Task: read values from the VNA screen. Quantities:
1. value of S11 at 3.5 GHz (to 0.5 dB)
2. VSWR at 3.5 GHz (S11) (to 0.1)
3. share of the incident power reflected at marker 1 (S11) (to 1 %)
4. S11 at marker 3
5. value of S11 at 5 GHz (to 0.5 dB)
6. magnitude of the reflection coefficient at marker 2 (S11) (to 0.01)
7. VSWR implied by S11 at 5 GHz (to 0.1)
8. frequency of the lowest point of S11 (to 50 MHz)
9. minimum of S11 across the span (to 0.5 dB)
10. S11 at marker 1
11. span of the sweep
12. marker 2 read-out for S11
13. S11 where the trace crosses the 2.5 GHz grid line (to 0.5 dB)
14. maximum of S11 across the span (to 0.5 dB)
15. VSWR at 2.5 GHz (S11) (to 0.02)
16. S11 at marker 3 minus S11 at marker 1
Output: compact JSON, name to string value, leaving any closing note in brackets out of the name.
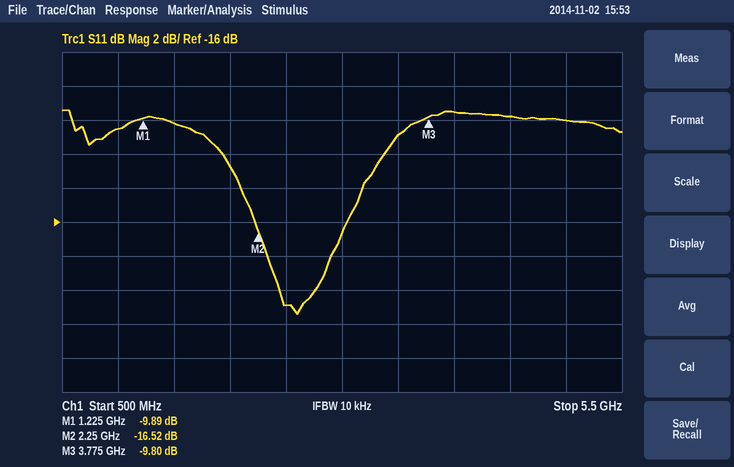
{"value of S11 at 3.5 GHz": "-11.0 dB", "VSWR at 3.5 GHz (S11)": "1.8", "share of the incident power reflected at marker 1 (S11)": "10 %", "S11 at marker 3": "-9.80 dB", "value of S11 at 5 GHz": "-10.0 dB", "magnitude of the reflection coefficient at marker 2 (S11)": "0.15", "VSWR implied by S11 at 5 GHz": "1.9", "frequency of the lowest point of S11": "2.60 GHz", "minimum of S11 across the span": "-21.5 dB", "S11 at marker 1": "-9.89 dB", "span of the sweep": "5 GHz", "marker 2 read-out for S11": "-16.52 dB", "S11 where the trace crosses the 2.5 GHz grid line": "-21.0 dB", "maximum of S11 across the span": "-9.5 dB", "VSWR at 2.5 GHz (S11)": "1.20", "S11 at marker 3 minus S11 at marker 1": "0.09 dB"}
